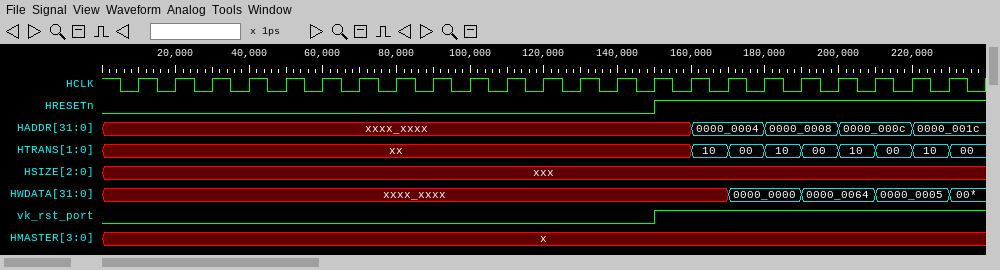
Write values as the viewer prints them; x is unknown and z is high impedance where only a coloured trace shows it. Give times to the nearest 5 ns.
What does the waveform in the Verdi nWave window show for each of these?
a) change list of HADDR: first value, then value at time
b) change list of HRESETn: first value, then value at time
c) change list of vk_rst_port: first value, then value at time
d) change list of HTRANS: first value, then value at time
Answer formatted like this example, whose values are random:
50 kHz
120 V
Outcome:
xxxx_xxxx, 0000_0004 at 160 ns, 0000_0008 at 180 ns, 0000_000c at 200 ns, 0000_001c at 220 ns
0, 1 at 150 ns
0, 1 at 150 ns
xx, 10 at 160 ns, 00 at 170 ns, 10 at 180 ns, 00 at 190 ns, 10 at 200 ns, 00 at 210 ns, 10 at 220 ns, 00 at 230 ns
